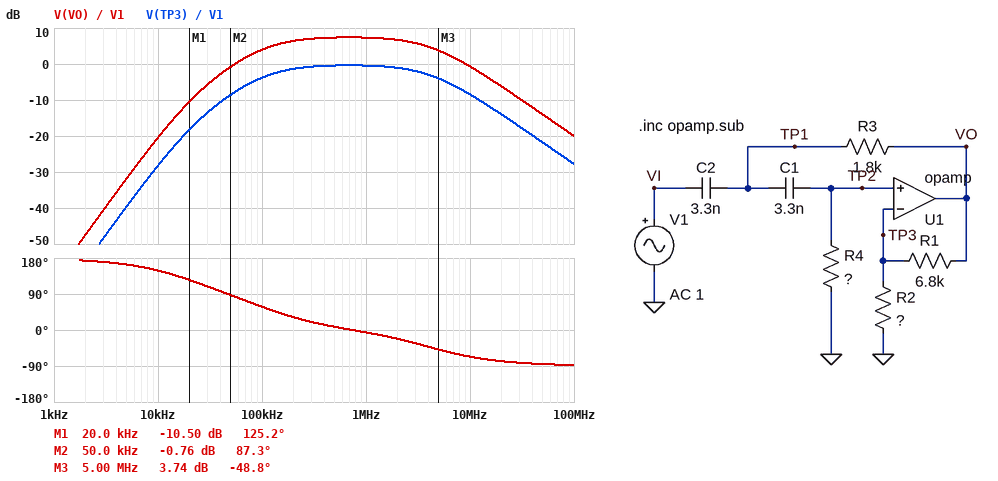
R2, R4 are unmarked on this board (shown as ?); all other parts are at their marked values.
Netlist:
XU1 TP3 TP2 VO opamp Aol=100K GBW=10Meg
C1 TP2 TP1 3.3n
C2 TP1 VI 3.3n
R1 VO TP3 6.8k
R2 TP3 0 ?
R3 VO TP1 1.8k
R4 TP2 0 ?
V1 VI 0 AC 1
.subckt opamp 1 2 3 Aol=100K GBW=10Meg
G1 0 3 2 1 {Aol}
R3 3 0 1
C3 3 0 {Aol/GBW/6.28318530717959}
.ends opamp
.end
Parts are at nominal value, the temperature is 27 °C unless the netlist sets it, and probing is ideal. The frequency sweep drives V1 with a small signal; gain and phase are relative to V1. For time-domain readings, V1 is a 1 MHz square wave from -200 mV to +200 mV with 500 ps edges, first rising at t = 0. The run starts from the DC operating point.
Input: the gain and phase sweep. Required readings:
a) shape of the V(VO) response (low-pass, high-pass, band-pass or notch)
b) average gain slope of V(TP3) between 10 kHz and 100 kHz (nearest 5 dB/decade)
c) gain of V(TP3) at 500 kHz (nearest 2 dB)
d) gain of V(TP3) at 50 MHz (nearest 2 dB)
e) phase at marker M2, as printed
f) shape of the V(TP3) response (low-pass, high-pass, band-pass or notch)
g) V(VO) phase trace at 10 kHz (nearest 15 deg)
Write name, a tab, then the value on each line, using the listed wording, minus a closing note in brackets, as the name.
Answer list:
shape of the V(VO) response	band-pass
average gain slope of V(TP3) between 10 kHz and 100 kHz	25 dB/decade
gain of V(TP3) at 500 kHz	0 dB
gain of V(TP3) at 50 MHz	-22 dB
phase at marker M2, as printed	87.3 deg
shape of the V(TP3) response	band-pass
V(VO) phase trace at 10 kHz	150 deg
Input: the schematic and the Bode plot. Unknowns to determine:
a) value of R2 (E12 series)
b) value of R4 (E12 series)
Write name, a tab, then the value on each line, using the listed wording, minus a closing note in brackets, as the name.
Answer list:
value of R2	4.7 kΩ
value of R4	560 Ω
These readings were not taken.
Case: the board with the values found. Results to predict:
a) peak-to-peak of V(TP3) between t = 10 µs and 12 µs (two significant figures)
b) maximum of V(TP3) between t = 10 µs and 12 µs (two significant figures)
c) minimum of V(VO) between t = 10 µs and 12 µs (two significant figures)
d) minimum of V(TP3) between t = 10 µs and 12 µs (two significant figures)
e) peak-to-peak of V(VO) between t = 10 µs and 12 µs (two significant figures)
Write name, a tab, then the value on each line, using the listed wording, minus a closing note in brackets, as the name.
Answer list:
peak-to-peak of V(TP3) between t = 10 µs and 12 µs	420 mV
maximum of V(TP3) between t = 10 µs and 12 µs	200 mV
minimum of V(VO) between t = 10 µs and 12 µs	-540 mV
minimum of V(TP3) between t = 10 µs and 12 µs	-220 mV
peak-to-peak of V(VO) between t = 10 µs and 12 µs	1.0 V
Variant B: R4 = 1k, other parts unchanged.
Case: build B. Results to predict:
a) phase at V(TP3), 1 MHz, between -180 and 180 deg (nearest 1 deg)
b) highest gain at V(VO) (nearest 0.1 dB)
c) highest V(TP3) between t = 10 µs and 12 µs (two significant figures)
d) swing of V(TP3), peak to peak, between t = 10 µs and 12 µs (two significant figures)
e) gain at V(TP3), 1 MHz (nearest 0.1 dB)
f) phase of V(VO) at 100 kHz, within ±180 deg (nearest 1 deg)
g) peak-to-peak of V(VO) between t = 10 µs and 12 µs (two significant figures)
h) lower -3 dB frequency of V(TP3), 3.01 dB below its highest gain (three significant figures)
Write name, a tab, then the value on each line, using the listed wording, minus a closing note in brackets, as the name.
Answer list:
phase at V(TP3), 1 MHz, between -180 and 180 deg	-10 deg
highest gain at V(VO)	7.6 dB
highest V(TP3) between t = 10 µs and 12 µs	170 mV
swing of V(TP3), peak to peak, between t = 10 µs and 12 µs	400 mV
gain at V(TP3), 1 MHz	-0.4 dB
phase of V(VO) at 100 kHz, within ±180 deg	32 deg
peak-to-peak of V(VO) between t = 10 µs and 12 µs	980 mV
lower -3 dB frequency of V(TP3), 3.01 dB below its highest gain	40.4 kHz
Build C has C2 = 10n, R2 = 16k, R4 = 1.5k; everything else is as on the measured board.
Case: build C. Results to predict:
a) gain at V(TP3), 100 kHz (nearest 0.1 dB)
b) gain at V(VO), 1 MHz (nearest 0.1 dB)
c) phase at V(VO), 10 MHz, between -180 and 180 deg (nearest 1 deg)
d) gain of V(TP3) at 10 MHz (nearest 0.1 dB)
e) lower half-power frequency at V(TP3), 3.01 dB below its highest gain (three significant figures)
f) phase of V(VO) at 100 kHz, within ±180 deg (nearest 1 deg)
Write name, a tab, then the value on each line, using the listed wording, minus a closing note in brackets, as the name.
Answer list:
gain at V(TP3), 100 kHz	-0.4 dB
gain at V(VO), 1 MHz	3.0 dB
phase at V(VO), 10 MHz, between -180 and 180 deg	-55 deg
gain of V(TP3) at 10 MHz	-4.8 dB
lower half-power frequency at V(TP3), 3.01 dB below its highest gain	31.8 kHz
phase of V(VO) at 100 kHz, within ±180 deg	21 deg
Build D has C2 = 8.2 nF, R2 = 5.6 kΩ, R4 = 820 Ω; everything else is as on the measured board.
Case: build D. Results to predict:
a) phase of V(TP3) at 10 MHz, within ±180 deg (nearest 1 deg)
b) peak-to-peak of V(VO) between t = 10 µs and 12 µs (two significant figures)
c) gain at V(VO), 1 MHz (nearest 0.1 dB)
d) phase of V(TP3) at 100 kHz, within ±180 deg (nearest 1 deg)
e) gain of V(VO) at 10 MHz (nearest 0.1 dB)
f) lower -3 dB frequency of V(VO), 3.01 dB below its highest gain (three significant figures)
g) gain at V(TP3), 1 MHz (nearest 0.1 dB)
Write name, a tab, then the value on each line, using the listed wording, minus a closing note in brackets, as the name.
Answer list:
phase of V(TP3) at 10 MHz, within ±180 deg	-65 deg
peak-to-peak of V(VO) between t = 10 µs and 12 µs	910 mV
gain at V(VO), 1 MHz	6.6 dB
phase of V(TP3) at 100 kHz, within ±180 deg	35 deg
gain of V(VO) at 10 MHz	-0.8 dB
lower -3 dB frequency of V(VO), 3.01 dB below its highest gain	58.6 kHz
gain at V(TP3), 1 MHz	-0.3 dB
